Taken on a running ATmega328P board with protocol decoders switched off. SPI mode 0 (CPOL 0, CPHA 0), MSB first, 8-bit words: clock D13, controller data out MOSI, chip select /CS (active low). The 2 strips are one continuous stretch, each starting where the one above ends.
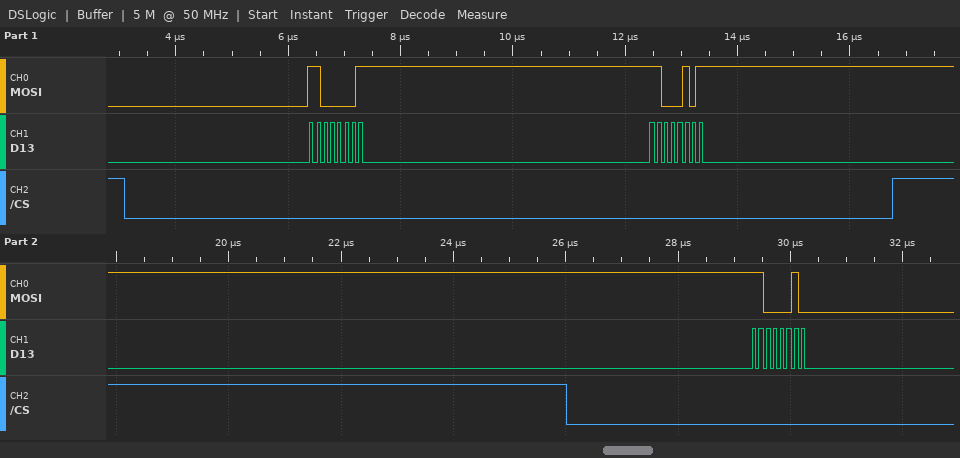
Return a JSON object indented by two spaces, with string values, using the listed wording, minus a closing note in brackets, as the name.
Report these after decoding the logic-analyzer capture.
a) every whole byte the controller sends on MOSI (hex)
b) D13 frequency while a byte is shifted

{
  "every whole byte the controller sends on MOSI": "C1 C5 C2",
  "D13 frequency while a byte is shifted": "8 MHz"
}
